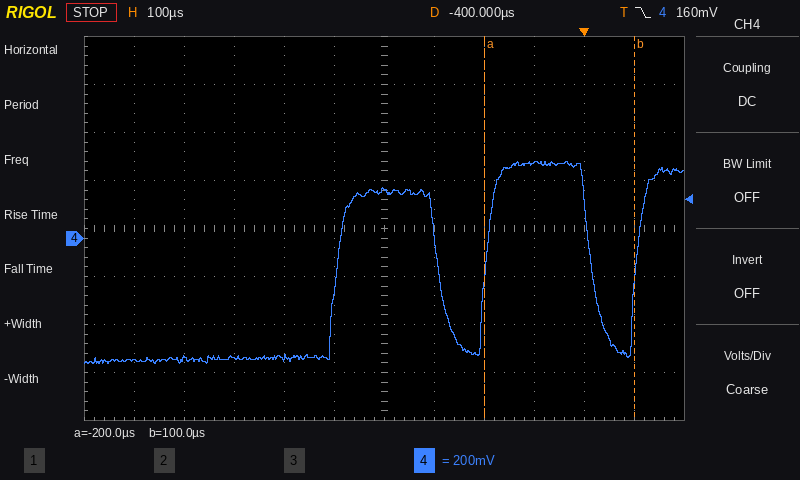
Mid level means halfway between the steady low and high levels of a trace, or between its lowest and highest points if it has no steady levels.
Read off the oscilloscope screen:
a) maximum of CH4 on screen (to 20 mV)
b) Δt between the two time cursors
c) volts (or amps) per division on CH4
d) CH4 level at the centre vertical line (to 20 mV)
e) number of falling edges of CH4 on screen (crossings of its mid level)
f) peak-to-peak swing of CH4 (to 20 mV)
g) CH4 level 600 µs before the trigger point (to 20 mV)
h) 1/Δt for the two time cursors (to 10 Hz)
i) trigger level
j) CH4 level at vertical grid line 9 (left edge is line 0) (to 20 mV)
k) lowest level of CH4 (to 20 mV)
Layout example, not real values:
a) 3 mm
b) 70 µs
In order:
a) 320 mV
b) 300 µs
c) 200 mV
d) 200 mV
e) 2
f) 840 mV
g) -500 mV
h) 3.33 kHz
i) 160 mV
j) 320 mV
k) -520 mV
